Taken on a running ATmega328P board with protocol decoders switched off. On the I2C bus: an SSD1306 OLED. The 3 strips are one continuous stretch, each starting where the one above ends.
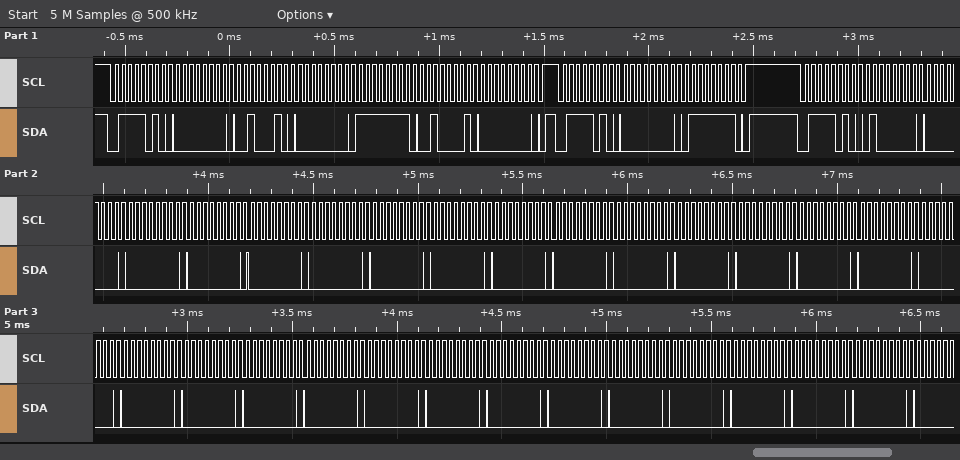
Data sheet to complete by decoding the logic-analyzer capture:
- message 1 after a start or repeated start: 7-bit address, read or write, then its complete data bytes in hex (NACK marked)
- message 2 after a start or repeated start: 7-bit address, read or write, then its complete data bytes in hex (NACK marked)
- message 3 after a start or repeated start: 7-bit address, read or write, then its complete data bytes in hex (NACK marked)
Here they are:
0x3D write: 00 22 00 FF 21 00
0x3D write: 00 7F
0x3D write: 40 00 00 00 00 00 00 00 00 00 00 00 00 00 00 00 00 00 00 00 00 00 00 00 00 00 00 00 00
